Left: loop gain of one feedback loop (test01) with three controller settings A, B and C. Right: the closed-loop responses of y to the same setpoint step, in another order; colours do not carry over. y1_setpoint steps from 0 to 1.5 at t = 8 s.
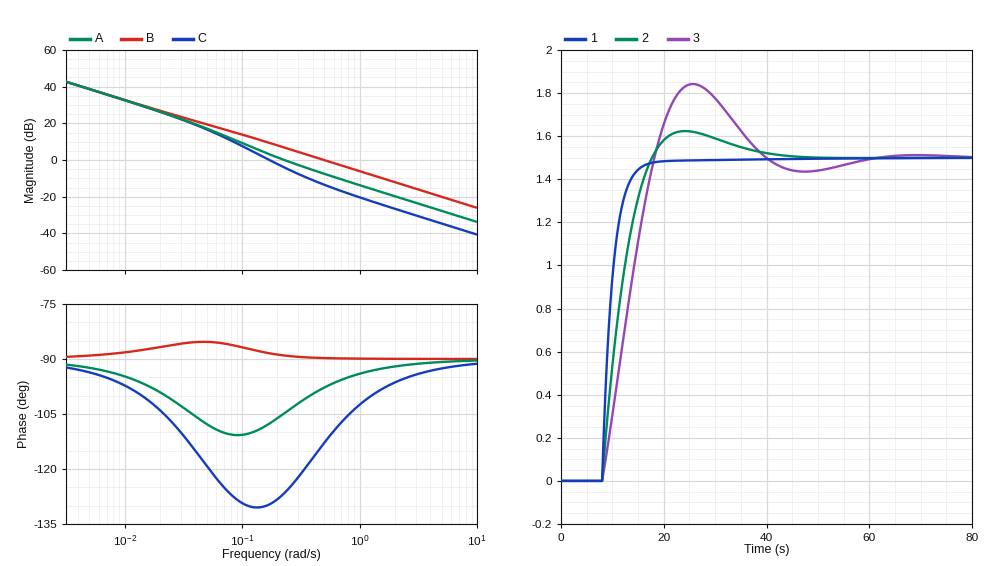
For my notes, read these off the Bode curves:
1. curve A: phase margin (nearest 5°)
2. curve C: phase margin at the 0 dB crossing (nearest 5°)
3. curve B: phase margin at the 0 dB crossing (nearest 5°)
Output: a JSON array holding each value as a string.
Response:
["75°", "50°", "90°"]
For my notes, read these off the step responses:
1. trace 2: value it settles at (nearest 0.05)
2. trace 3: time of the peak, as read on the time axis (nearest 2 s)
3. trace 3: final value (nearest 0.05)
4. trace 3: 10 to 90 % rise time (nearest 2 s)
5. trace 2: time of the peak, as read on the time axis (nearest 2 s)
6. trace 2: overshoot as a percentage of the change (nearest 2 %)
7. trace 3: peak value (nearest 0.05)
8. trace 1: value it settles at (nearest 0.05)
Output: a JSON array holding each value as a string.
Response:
["1.50", "26 s", "1.50", "8 s", "24 s", "8 %", "1.85", "1.50"]
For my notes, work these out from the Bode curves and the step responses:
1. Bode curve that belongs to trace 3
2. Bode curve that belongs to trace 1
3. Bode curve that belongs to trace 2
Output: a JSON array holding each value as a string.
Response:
["C", "B", "A"]
